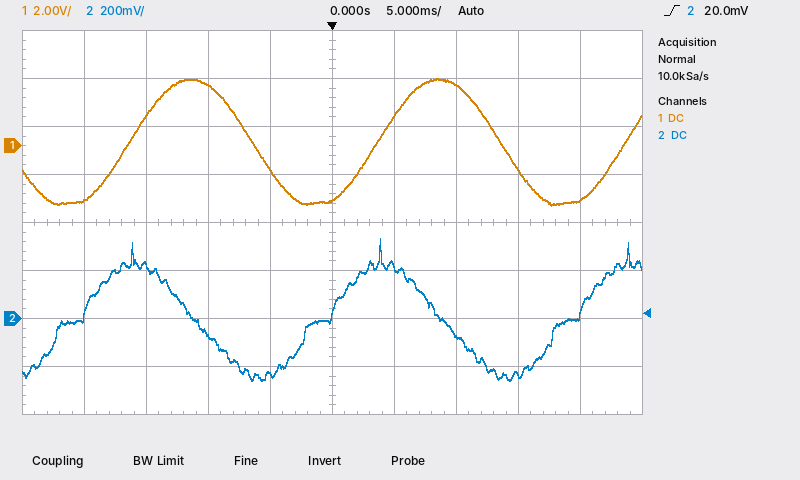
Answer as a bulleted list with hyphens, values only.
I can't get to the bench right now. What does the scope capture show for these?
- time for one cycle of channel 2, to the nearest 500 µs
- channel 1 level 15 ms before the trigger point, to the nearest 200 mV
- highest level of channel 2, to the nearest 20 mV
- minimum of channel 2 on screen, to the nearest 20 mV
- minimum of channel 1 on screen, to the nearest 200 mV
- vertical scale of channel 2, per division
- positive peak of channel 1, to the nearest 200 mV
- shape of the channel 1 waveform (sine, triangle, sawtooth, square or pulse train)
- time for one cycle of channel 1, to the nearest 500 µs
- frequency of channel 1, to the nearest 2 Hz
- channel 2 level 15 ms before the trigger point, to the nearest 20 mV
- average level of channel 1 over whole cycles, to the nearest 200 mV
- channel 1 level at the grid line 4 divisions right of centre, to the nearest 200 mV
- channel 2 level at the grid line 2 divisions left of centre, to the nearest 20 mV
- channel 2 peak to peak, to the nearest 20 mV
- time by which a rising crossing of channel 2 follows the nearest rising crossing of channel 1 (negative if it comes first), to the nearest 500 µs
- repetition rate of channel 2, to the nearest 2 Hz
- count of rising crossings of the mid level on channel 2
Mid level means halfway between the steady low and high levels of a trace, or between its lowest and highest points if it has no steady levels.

- 20.0 ms
- 1.2 V
- 340 mV
- -260 mV
- -2.4 V
- 200 mV
- 2.8 V
- sine
- 20.0 ms
- 50 Hz
- 220 mV
- 200 mV
- -2.2 V
- -60 mV
- 600 mV
- -3.5 ms
- 50 Hz
- 3
